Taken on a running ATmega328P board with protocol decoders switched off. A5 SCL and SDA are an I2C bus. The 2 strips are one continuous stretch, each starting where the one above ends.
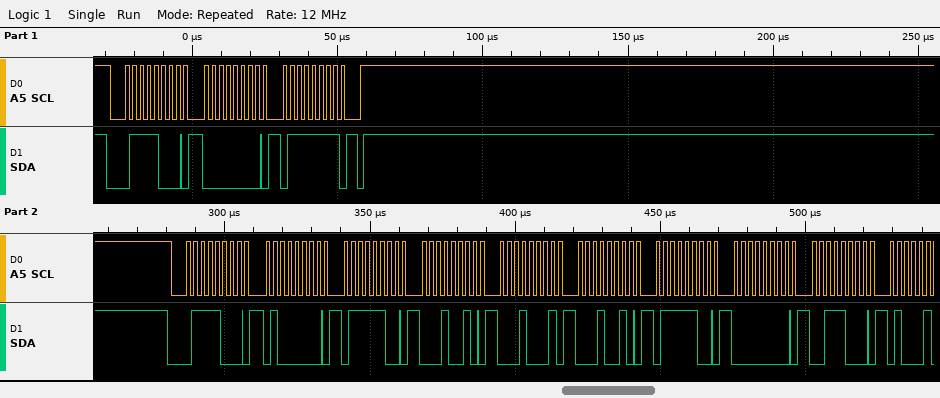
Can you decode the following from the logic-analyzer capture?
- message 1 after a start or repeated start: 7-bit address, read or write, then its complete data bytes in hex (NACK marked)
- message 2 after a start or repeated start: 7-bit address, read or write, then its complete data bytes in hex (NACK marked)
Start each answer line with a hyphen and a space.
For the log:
- 0x3C write: 00 7F
- 0x3C write: 40 7C 12 11 12 7C 00 38
